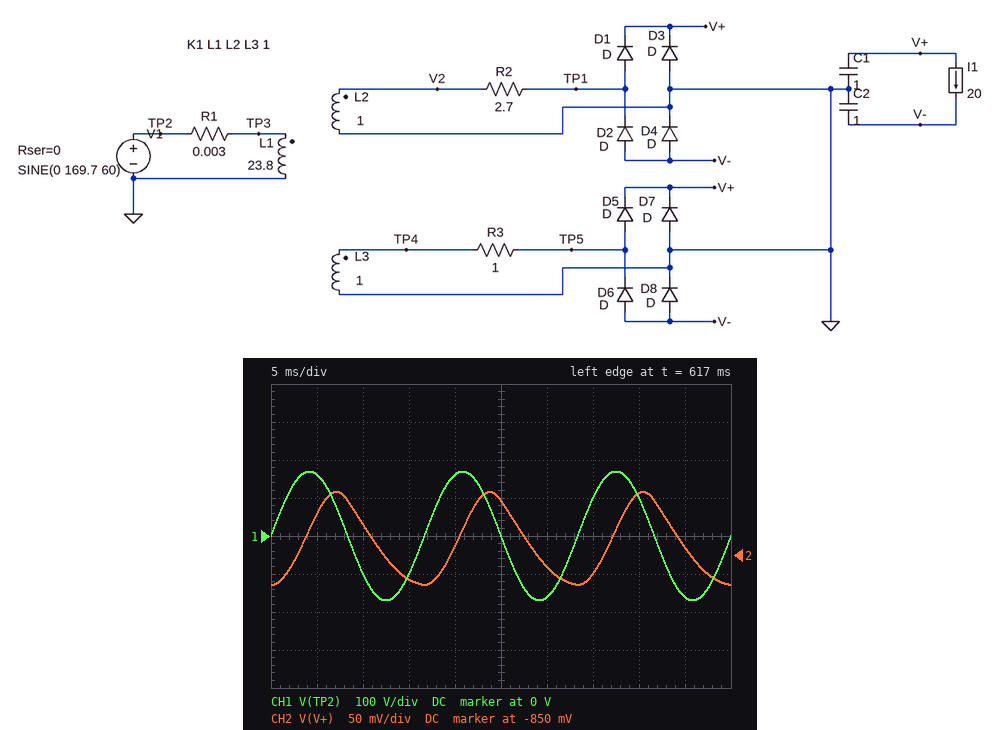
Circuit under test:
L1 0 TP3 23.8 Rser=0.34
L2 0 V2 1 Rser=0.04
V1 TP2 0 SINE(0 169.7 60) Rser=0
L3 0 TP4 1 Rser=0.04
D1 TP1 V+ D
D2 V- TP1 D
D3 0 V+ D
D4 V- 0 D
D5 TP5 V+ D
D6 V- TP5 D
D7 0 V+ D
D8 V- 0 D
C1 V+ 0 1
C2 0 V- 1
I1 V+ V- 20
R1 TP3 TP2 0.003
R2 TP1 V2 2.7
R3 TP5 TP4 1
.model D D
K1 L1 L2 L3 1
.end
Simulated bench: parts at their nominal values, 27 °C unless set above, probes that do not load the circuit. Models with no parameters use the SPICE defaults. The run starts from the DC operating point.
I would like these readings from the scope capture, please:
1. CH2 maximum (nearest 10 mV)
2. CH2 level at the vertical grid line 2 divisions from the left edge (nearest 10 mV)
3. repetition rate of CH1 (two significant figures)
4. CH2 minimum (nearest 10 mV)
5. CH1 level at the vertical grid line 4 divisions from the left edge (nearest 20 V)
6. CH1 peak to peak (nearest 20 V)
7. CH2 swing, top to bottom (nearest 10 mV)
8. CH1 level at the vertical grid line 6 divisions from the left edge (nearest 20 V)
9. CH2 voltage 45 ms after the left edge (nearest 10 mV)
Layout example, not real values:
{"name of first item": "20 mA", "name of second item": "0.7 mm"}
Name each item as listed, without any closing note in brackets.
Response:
{"CH2 maximum": "-770 mV", "CH2 level at the vertical grid line 2 divisions from the left edge": "-810 mV", "repetition rate of CH1": "60 Hz", "CH2 minimum": "-890 mV", "CH1 level at the vertical grid line 4 divisions from the left edge": "160 V", "CH1 peak to peak": "340 V", "CH2 swing, top to bottom": "120 mV", "CH1 level at the vertical grid line 6 divisions from the left edge": "-160 V", "CH2 voltage 45 ms after the left edge": "-840 mV"}
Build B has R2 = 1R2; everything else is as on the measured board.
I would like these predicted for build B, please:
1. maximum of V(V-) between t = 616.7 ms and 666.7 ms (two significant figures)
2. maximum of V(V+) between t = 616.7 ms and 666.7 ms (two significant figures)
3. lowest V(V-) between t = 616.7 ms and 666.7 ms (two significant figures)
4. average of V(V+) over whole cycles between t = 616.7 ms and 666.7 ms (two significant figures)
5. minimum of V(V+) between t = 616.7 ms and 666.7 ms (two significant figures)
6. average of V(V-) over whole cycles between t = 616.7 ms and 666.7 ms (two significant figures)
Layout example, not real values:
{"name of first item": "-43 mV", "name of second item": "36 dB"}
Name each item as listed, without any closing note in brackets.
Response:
{"maximum of V(V-) between t = 616.7 ms and 666.7 ms": "860 mV", "maximum of V(V+) between t = 616.7 ms and 666.7 ms": "-680 mV", "lowest V(V-) between t = 616.7 ms and 666.7 ms": "680 mV", "average of V(V+) over whole cycles between t = 616.7 ms and 666.7 ms": "-770 mV", "minimum of V(V+) between t = 616.7 ms and 666.7 ms": "-860 mV", "average of V(V-) over whole cycles between t = 616.7 ms and 666.7 ms": "770 mV"}
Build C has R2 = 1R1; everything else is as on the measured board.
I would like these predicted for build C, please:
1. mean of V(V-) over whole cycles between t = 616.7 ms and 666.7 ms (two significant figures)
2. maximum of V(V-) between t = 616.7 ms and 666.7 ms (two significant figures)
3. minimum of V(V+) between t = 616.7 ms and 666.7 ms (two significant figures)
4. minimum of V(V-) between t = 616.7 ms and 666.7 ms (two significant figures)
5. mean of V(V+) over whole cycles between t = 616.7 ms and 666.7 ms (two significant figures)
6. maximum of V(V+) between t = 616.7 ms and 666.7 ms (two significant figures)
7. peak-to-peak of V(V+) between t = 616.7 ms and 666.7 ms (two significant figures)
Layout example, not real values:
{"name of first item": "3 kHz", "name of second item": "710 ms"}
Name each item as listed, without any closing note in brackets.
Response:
{"mean of V(V-) over whole cycles between t = 616.7 ms and 666.7 ms": "740 mV", "maximum of V(V-) between t = 616.7 ms and 666.7 ms": "830 mV", "minimum of V(V+) between t = 616.7 ms and 666.7 ms": "-830 mV", "minimum of V(V-) between t = 616.7 ms and 666.7 ms": "650 mV", "mean of V(V+) over whole cycles between t = 616.7 ms and 666.7 ms": "-740 mV", "maximum of V(V+) between t = 616.7 ms and 666.7 ms": "-650 mV", "peak-to-peak of V(V+) between t = 616.7 ms and 666.7 ms": "180 mV"}
